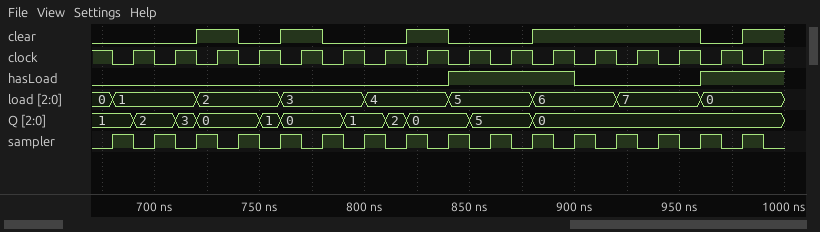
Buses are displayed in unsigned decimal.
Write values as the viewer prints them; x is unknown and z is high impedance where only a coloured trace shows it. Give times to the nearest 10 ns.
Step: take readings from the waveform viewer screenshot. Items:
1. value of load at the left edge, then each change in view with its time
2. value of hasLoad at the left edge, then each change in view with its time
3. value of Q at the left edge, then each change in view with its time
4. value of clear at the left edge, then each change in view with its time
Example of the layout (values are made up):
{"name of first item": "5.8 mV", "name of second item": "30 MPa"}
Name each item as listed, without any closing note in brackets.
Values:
{"value of load at the left edge, then each change in view with its time": "0, 1 at 680 ns, 2 at 720 ns, 3 at 760 ns, 4 at 800 ns, 5 at 840 ns, 6 at 880 ns, 7 at 920 ns, 0 at 960 ns", "value of hasLoad at the left edge, then each change in view with its time": "0, 1 at 840 ns, 0 at 900 ns, 1 at 960 ns", "value of Q at the left edge, then each change in view with its time": "1, 2 at 690 ns, 3 at 710 ns, 0 at 720 ns, 1 at 750 ns, 0 at 760 ns, 1 at 790 ns, 2 at 810 ns, 0 at 820 ns, 5 at 850 ns, 0 at 880 ns", "value of clear at the left edge, then each change in view with its time": "0, 1 at 720 ns, 0 at 740 ns, 1 at 760 ns, 0 at 780 ns, 1 at 820 ns, 0 at 840 ns, 1 at 880 ns, 0 at 960 ns, 1 at 980 ns"}
